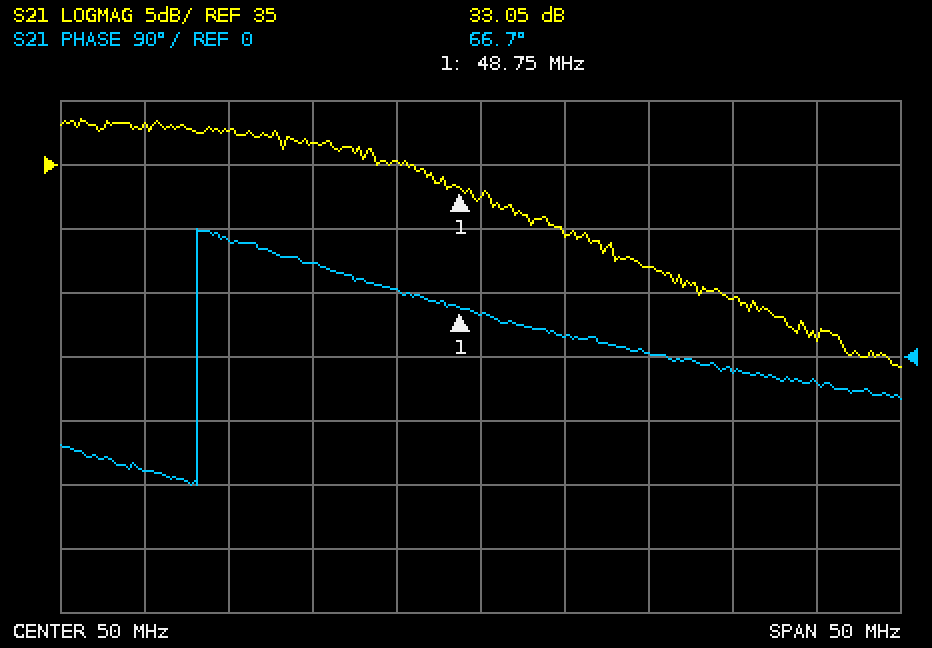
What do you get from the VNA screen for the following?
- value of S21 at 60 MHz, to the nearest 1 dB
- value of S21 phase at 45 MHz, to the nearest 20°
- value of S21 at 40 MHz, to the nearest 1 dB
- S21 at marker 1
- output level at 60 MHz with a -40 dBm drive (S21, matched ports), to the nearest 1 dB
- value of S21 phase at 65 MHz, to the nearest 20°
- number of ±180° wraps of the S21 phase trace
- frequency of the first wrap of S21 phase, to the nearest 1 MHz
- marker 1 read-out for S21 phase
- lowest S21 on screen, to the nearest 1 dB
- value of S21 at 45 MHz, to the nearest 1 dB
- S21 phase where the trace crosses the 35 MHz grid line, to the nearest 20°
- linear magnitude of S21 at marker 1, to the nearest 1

27 dB
100°
37 dB
33.05 dB
-13 dBm
-20°
1
33 MHz
66.7°
19 dB
35 dB
160°
45
